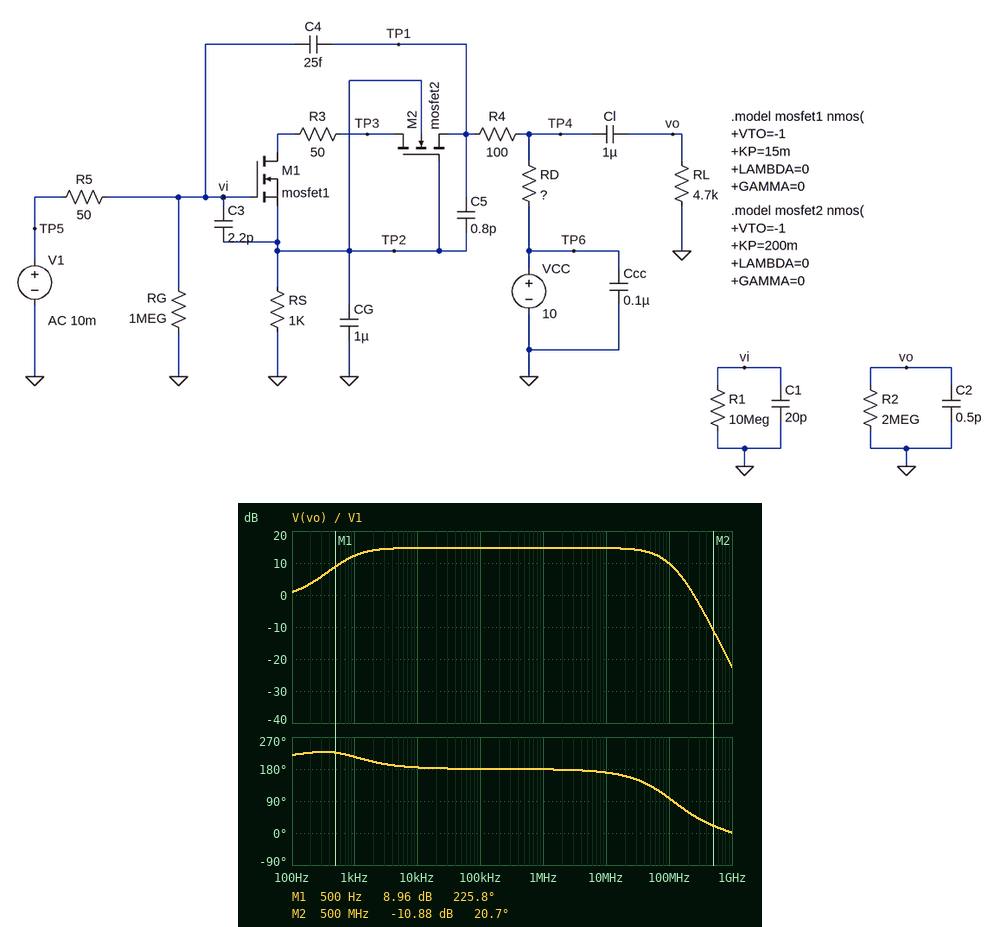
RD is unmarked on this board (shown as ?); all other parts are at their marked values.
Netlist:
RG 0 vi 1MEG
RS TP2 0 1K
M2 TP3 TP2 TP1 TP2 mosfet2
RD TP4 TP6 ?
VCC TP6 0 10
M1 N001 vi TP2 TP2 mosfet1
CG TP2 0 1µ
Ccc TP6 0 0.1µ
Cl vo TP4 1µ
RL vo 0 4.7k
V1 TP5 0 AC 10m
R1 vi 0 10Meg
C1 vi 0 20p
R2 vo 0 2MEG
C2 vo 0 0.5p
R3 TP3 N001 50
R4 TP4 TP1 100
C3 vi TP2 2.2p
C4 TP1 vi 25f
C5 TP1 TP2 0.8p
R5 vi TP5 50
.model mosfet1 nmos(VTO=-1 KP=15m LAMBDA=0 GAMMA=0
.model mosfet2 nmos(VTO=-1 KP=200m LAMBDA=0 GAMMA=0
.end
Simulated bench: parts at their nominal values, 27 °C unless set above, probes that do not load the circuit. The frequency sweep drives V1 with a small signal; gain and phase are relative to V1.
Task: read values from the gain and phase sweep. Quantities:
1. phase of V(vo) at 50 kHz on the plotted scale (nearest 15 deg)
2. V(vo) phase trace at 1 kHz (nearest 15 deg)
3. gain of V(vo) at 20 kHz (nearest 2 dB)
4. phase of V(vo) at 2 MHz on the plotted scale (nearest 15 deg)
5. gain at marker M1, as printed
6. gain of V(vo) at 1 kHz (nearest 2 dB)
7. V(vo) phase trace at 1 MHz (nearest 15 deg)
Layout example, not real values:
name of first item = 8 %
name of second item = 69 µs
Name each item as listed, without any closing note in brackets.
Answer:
phase of V(vo) at 50 kHz on the plotted scale = 180 deg
V(vo) phase trace at 1 kHz = 210 deg
gain of V(vo) at 20 kHz = 14 dB
phase of V(vo) at 2 MHz on the plotted scale = 180 deg
gain at marker M1, as printed = 8.96 dB
gain of V(vo) at 1 kHz = 12 dB
V(vo) phase trace at 1 MHz = 180 deg
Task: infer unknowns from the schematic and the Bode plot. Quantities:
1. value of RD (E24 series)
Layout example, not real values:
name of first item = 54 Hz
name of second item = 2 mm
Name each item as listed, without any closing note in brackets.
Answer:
value of RD = 1.6 kΩ
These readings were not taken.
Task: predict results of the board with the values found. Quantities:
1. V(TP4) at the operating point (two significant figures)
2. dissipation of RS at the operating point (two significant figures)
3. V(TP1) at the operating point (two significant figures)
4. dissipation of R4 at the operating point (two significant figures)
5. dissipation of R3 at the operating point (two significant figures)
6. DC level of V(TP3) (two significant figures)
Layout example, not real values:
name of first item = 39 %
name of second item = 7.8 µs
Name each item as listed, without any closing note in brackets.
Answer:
V(TP4) at the operating point = 8.9 V
dissipation of RS at the operating point = 480 µW
V(TP1) at the operating point = 8.8 V
dissipation of R4 at the operating point = 48 µW
dissipation of R3 at the operating point = 24 µW
DC level of V(TP3) = 1.6 V
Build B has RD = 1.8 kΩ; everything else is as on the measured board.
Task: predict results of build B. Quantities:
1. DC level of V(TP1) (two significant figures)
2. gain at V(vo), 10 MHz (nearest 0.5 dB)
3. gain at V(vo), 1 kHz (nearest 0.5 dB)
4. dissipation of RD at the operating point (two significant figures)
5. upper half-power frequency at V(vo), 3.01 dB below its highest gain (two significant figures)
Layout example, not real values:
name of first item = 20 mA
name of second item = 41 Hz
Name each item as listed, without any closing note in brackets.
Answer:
DC level of V(TP1) = 8.7 V
gain at V(vo), 10 MHz = 15.5 dB
gain at V(vo), 1 kHz = 13.0 dB
dissipation of RD at the operating point = 870 µW
upper half-power frequency at V(vo), 3.01 dB below its highest gain = 70 MHz
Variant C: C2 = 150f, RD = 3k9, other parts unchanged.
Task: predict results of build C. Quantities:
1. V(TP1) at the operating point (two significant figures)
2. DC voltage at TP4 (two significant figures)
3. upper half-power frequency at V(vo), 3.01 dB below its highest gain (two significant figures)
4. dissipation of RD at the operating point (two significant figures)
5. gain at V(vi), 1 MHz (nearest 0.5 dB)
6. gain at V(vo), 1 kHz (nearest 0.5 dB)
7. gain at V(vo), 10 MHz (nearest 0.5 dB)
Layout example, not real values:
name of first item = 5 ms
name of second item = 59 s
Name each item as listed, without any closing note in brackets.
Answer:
V(TP1) at the operating point = 7.2 V
DC voltage at TP4 = 7.3 V
upper half-power frequency at V(vo), 3.01 dB below its highest gain = 61 MHz
dissipation of RD at the operating point = 1.9 mW
gain at V(vi), 1 MHz = 0 dB
gain at V(vo), 1 kHz = 17.5 dB
gain at V(vo), 10 MHz = 19.5 dB
